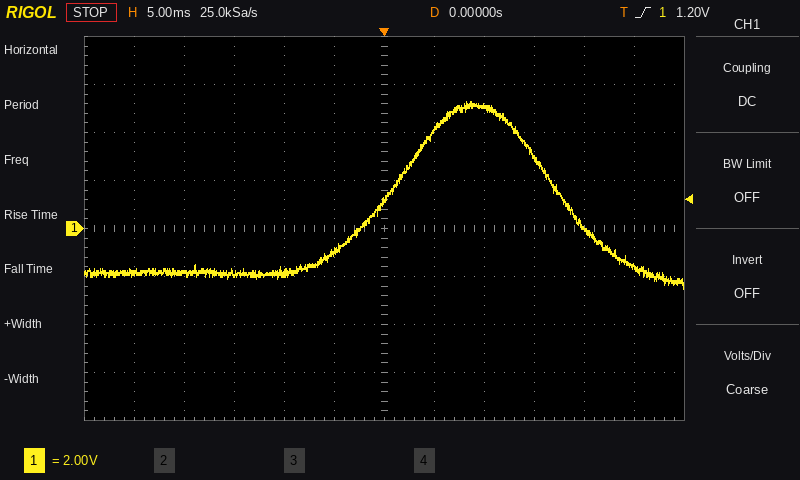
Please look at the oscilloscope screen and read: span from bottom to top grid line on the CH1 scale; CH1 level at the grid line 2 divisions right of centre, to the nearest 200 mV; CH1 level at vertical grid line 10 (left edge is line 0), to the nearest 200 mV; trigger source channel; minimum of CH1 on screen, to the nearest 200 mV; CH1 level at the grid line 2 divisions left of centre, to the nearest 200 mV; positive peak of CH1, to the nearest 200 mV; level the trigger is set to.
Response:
16 V
5.0 V
0.0 V
CH1
-2.4 V
-1.8 V
5.2 V
1.20 V
